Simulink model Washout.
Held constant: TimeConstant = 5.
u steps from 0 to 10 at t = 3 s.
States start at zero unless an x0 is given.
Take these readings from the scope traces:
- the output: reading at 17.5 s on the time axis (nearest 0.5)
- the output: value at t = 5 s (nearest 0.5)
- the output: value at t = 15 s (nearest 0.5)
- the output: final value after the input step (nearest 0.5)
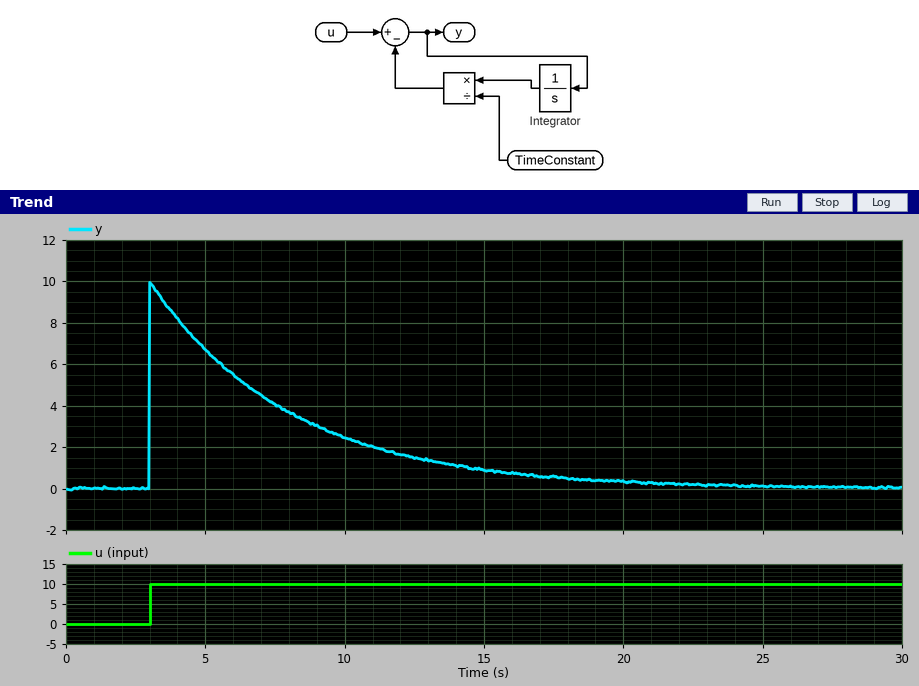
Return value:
0.5
6.5
1.0
0.0
